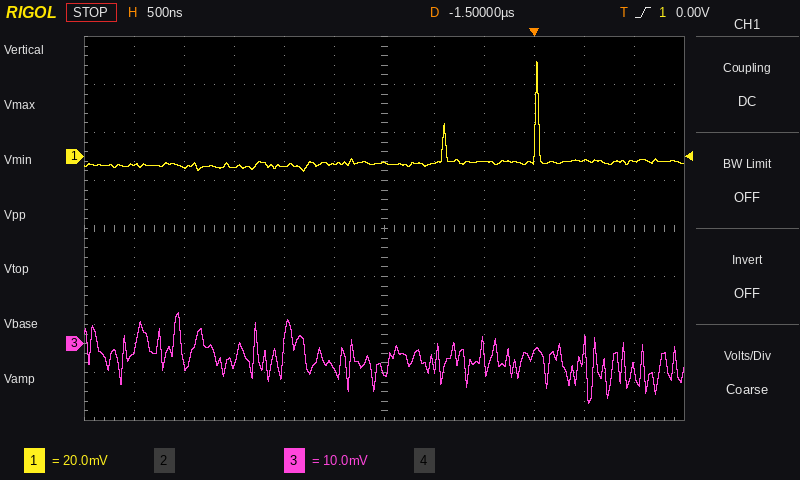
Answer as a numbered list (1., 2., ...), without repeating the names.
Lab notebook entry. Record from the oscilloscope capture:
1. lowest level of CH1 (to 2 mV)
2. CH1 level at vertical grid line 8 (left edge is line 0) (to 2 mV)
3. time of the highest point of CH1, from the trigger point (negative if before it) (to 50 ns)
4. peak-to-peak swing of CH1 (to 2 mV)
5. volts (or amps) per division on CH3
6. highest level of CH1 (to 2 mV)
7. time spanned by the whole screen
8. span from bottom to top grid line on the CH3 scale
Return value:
1. -6 mV
2. -2 mV
3. +50 ns
4. 46 mV
5. 10 mV
6. 40 mV
7. 6 µs
8. 80 mV
